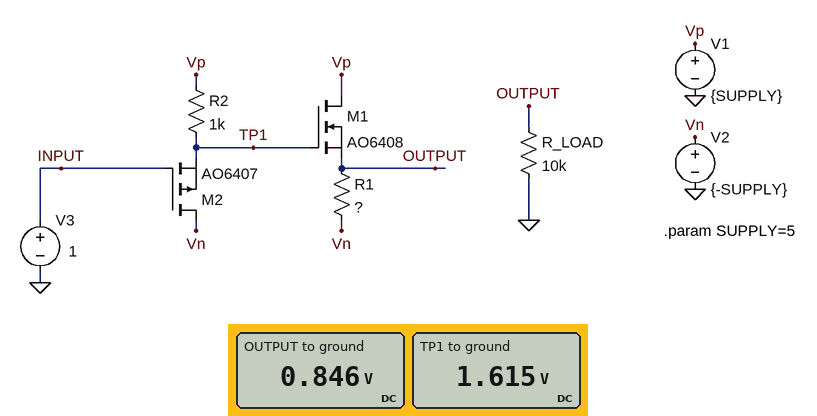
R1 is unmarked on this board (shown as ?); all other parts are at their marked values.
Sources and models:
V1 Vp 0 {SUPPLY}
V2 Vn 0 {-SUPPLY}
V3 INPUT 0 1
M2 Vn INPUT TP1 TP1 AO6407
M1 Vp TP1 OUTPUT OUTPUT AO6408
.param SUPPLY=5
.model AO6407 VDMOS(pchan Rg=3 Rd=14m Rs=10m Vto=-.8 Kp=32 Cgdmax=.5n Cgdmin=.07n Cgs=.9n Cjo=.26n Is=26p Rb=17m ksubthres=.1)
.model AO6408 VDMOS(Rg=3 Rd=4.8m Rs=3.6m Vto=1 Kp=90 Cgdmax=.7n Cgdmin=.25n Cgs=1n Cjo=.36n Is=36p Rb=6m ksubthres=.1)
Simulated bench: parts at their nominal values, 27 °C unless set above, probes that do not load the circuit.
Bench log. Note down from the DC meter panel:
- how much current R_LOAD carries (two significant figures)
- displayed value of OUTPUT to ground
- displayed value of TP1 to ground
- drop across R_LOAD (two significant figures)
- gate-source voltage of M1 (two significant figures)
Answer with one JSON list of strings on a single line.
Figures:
["85 µA", "0.846 V", "1.615 V", "850 mV", "770 mV"]
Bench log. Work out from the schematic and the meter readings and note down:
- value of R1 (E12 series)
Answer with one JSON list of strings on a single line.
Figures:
["1.5 kΩ"]
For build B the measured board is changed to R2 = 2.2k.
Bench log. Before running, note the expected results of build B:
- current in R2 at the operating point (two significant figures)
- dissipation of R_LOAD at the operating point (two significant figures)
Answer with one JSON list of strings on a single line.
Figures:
["1.6 mA", "65 µW"]
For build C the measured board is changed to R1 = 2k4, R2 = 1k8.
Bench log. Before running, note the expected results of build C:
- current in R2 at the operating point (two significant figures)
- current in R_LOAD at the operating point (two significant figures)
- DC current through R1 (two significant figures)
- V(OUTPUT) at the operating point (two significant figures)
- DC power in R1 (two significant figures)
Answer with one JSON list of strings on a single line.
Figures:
["1.9 mA", "84 µA", "2.4 mA", "840 mV", "14 mW"]
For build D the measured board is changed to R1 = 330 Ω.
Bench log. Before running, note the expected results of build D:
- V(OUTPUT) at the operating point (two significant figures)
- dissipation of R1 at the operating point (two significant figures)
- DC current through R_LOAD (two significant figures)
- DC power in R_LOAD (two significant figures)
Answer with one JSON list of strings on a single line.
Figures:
["770 mV", "100 mW", "77 µA", "59 µW"]
